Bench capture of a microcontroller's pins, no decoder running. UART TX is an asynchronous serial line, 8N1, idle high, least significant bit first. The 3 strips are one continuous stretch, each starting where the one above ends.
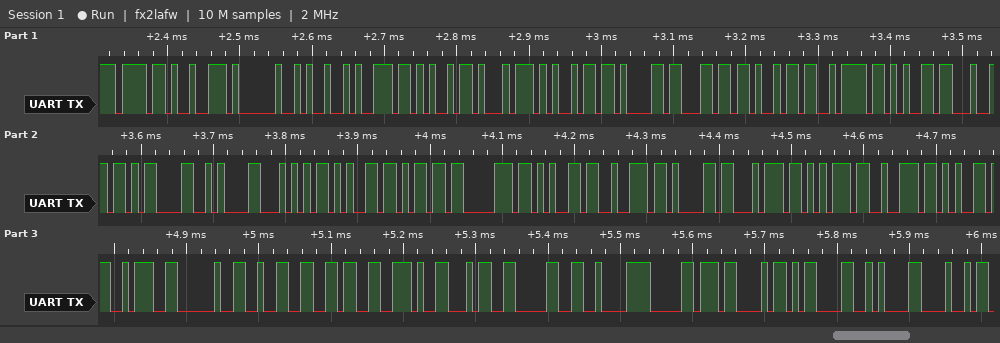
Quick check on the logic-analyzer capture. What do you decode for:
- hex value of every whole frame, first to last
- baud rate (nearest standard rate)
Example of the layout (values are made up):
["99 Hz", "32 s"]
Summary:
["0x6F 0x72 0x20 0x49 0x6E 0x69 0x74 0x69 0x61 0x6C 0x69 0x7A 0x65 0x64 0x0D 0x0A 0x54 0x65 0x6D 0x70 0x65 0x72 0x61 0x74 0x75 0x72 0x65 0x3A 0x20 0x32 0x36 0x2E 0x34 0x30 0xC2 0xB0 0x43 0x0D 0x0A 0x48", "115200 baud"]
